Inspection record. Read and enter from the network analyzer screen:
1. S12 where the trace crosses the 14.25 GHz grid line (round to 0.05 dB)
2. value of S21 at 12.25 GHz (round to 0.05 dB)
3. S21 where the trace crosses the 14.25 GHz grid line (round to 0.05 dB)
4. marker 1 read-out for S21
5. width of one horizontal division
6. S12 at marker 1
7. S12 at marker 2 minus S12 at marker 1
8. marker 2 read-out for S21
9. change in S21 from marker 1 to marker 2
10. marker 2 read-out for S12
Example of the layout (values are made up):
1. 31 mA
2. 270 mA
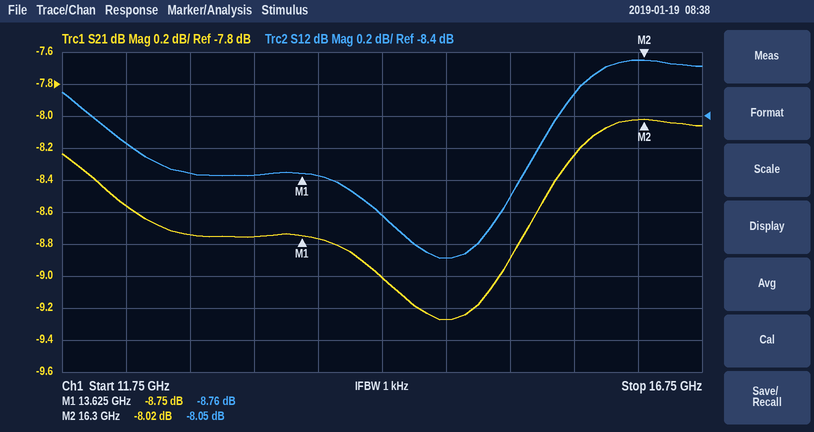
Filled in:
1. -9.00 dB
2. -8.55 dB
3. -9.00 dB
4. -8.75 dB
5. 500 MHz
6. -8.76 dB
7. 0.71 dB
8. -8.02 dB
9. 0.73 dB
10. -8.05 dB
